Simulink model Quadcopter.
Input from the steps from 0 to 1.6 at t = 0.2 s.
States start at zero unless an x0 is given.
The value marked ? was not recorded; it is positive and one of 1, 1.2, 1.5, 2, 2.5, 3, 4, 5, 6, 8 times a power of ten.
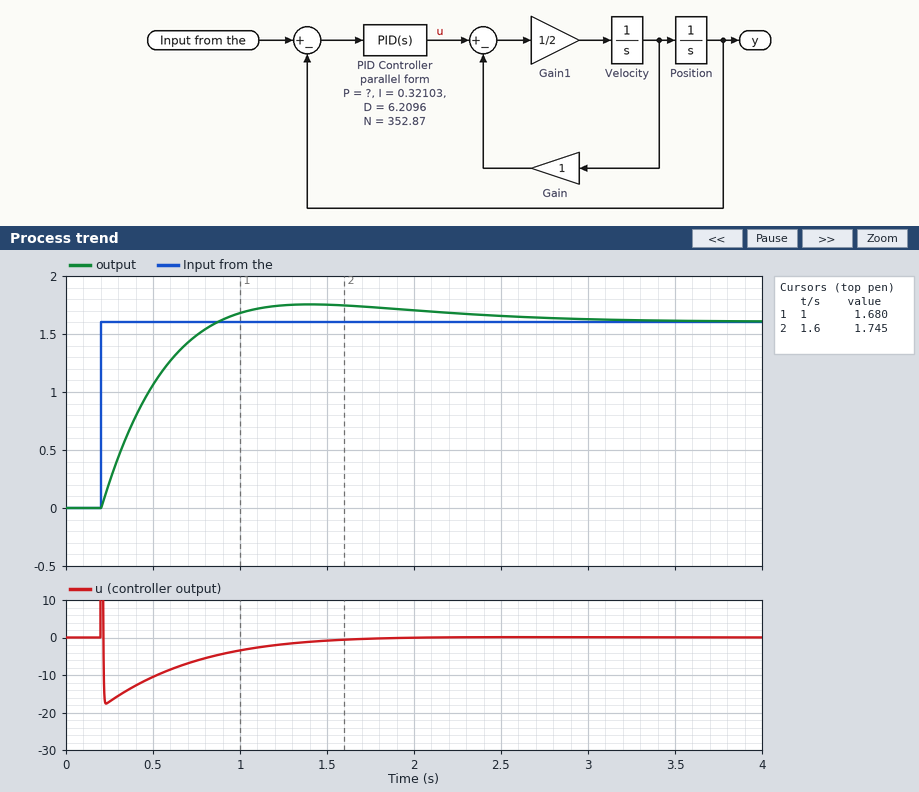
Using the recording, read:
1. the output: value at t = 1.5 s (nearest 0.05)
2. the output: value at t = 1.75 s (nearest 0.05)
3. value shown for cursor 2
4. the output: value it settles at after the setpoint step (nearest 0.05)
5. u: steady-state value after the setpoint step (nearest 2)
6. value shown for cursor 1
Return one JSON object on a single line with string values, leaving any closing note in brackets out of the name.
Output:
{"the output: value at t = 1.5 s": "1.75", "the output: value at t = 1.75 s": "1.75", "value shown for cursor 2": "1.745", "the output: value it settles at after the setpoint step": "1.60", "u: steady-state value after the setpoint step": "0", "value shown for cursor 1": "1.680"}
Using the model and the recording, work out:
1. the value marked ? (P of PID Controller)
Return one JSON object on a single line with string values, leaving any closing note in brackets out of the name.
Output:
{"the value marked ?": "8"}
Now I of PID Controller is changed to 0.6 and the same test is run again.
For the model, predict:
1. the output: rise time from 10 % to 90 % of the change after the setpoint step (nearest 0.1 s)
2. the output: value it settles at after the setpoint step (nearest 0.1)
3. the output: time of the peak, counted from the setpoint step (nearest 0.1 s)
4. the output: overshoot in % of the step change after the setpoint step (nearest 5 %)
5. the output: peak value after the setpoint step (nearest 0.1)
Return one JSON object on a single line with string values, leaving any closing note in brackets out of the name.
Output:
{"the output: rise time from 10 % to 90 % of the change after the setpoint step": "0.5 s", "the output: value it settles at after the setpoint step": "1.6", "the output: time of the peak, counted from the setpoint step": "1.2 s", "the output: overshoot in % of the step change after the setpoint step": "10 %", "the output: peak value after the setpoint step": "1.8"}
